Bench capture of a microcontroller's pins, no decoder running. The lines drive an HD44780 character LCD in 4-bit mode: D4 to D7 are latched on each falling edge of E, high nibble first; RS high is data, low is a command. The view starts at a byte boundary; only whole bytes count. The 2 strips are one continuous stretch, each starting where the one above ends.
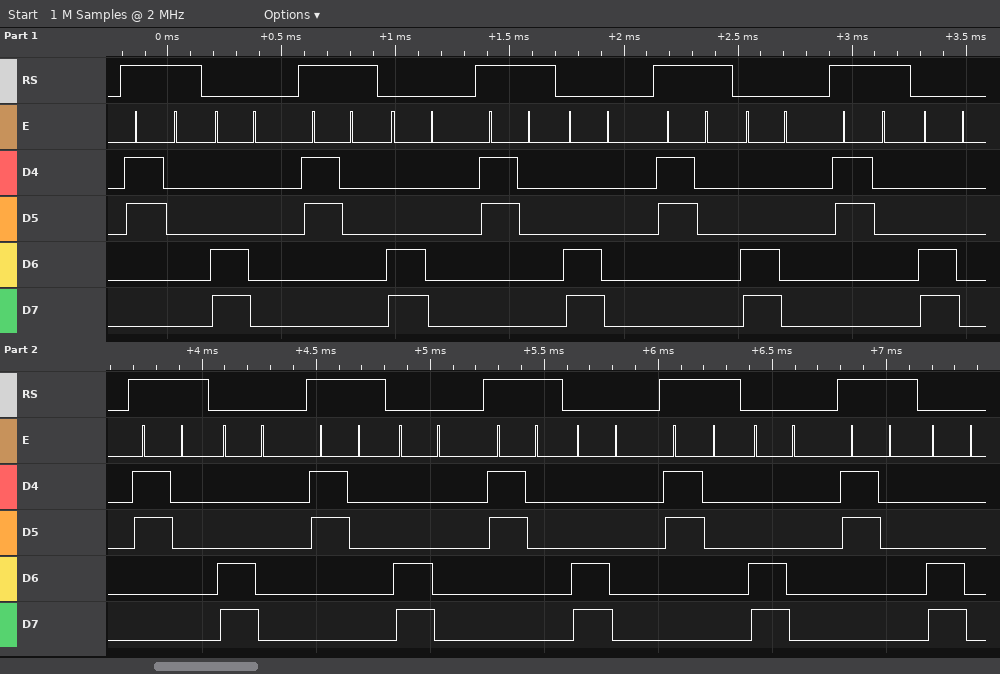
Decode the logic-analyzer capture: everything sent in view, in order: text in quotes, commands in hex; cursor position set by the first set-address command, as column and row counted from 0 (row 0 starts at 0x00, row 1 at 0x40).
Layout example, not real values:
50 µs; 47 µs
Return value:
"0" 0xC0 "0" 0xC0 "0" 0xC0 "0" 0xC0 "0" 0xC0 "0" 0xC0 "0" 0xC0 "0" 0xC0 "0" 0xC0 "0" 0xC0; column 0, row 1
